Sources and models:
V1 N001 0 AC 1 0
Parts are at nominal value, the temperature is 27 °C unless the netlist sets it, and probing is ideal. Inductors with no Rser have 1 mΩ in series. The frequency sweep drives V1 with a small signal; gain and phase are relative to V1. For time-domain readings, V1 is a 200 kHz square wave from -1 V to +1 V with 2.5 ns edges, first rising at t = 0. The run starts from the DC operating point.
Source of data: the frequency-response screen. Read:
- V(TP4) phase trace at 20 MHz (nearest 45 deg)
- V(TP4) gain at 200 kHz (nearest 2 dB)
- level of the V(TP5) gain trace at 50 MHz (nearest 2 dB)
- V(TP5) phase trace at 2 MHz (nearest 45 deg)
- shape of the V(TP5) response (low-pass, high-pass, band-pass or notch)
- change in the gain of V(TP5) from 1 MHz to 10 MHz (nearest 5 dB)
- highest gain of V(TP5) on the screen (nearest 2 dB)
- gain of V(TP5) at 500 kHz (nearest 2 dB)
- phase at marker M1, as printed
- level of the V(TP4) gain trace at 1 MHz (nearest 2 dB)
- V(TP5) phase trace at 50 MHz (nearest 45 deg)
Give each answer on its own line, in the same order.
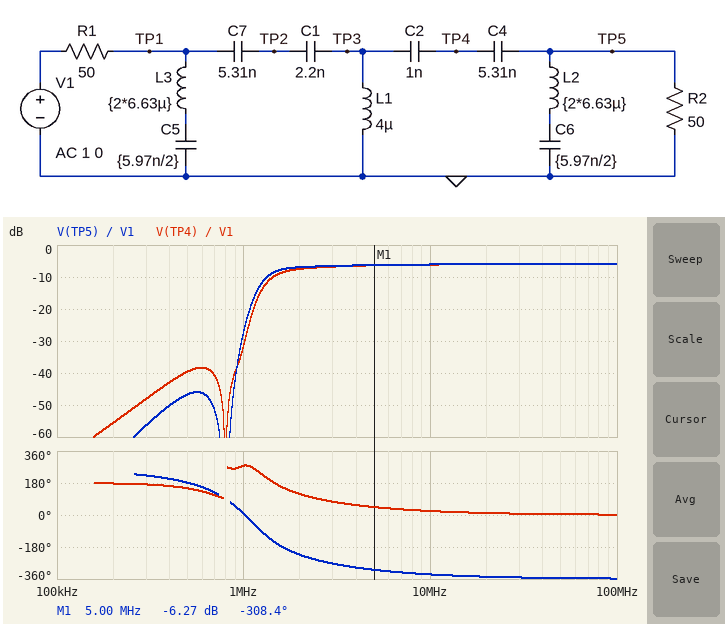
0 deg
-56 dB
-6 dB
-225 deg
high-pass
20 dB
-6 dB
-46 dB
-308.4 deg
-32 dB
-360 deg
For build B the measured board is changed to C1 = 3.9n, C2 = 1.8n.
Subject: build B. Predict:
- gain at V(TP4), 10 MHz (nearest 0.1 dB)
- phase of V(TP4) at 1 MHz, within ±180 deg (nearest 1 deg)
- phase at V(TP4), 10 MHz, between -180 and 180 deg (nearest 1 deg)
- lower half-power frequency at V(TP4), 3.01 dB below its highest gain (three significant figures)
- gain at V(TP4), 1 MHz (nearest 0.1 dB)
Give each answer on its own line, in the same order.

-6.0 dB
-117 deg
17 deg
1.31 MHz
-17.7 dB
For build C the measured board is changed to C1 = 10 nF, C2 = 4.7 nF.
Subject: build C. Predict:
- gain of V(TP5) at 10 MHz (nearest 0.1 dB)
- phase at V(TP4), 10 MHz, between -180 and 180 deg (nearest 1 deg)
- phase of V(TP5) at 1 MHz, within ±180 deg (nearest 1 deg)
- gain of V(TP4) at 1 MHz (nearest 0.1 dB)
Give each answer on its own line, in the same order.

-6.0 dB
12 deg
-138 deg
-12.6 dB
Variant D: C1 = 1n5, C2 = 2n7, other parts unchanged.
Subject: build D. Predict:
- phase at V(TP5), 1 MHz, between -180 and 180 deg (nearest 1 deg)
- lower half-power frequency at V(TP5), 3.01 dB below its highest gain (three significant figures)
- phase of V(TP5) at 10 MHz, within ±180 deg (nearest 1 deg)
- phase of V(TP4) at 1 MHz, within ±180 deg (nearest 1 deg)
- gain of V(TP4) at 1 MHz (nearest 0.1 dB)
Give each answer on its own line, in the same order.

-3 deg
1.17 MHz
22 deg
-93 deg
-24.6 dB
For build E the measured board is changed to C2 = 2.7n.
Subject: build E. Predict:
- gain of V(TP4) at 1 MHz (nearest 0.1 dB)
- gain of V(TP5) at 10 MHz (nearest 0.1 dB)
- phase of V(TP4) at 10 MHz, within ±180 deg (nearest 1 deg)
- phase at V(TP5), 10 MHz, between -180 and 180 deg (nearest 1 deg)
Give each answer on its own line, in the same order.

-19.9 dB
-6.0 dB
17 deg
20 deg
